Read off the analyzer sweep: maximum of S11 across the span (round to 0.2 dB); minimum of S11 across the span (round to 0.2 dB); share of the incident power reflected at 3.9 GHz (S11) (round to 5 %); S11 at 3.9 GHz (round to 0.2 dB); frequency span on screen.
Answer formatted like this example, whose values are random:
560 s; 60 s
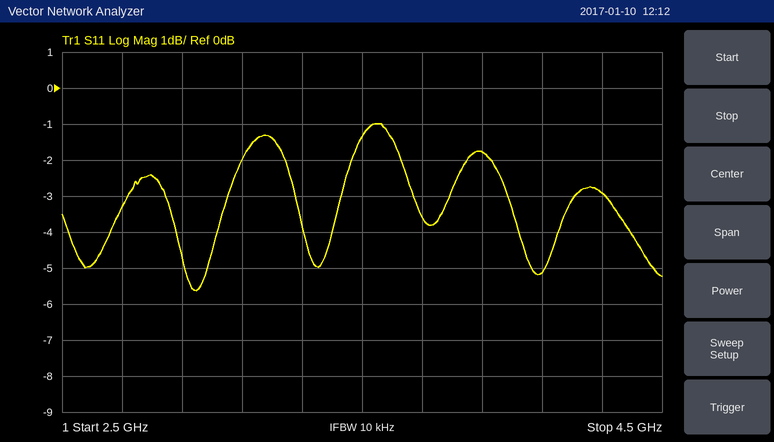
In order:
-1.0 dB; -5.6 dB; 65 %; -1.8 dB; 2 GHz
